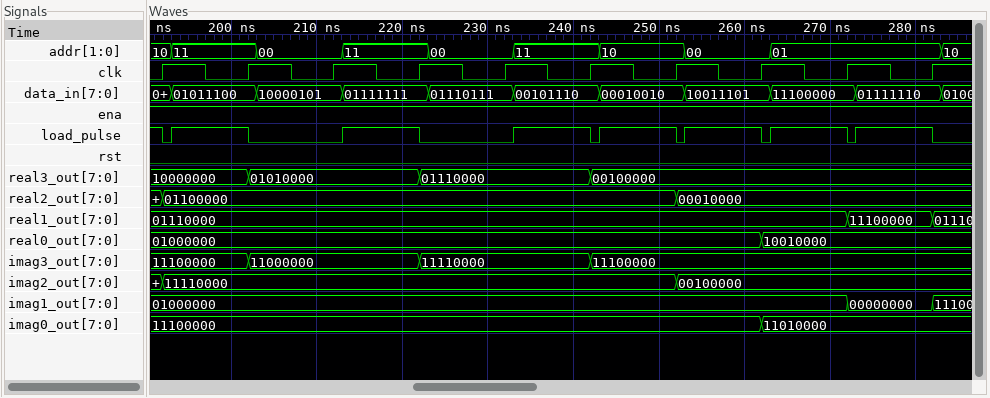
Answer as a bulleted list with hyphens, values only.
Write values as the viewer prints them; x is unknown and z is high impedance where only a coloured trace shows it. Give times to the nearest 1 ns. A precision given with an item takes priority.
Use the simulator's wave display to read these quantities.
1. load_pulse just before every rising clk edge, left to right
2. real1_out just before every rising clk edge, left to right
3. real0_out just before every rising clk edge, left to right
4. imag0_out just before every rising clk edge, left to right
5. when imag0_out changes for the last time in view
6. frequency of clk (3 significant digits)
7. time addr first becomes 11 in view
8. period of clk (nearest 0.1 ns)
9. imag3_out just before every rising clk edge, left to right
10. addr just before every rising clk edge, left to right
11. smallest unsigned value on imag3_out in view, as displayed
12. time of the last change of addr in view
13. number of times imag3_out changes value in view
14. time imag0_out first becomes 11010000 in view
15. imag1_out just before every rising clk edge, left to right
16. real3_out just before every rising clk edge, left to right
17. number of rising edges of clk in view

- 1 1 0 1 0 1 1 1 1 1
- 01110000, 01110000, 01110000, 01110000, 01110000, 01110000, 01110000, 01110000, 01110000, 11100000
- 01000000, 01000000, 01000000, 01000000, 01000000, 01000000, 01000000, 01000000, 10010000, 10010000
- 11100000, 11100000, 11100000, 11100000, 11100000, 11100000, 11100000, 11100000, 11010000, 11010000
- 262 ns
- 100 MHz
- 193 ns
- 10 ns
- 11100000, 11100000, 11000000, 11000000, 11110000, 11110000, 11100000, 11100000, 11100000, 11100000
- 10, 11, 00, 11, 00, 11, 10, 00, 01, 01
- 11000000
- 283 ns
- 3
- 262 ns
- 01000000, 01000000, 01000000, 01000000, 01000000, 01000000, 01000000, 01000000, 01000000, 00000000
- 10000000, 10000000, 01010000, 01010000, 01110000, 01110000, 00100000, 00100000, 00100000, 00100000
- 10
